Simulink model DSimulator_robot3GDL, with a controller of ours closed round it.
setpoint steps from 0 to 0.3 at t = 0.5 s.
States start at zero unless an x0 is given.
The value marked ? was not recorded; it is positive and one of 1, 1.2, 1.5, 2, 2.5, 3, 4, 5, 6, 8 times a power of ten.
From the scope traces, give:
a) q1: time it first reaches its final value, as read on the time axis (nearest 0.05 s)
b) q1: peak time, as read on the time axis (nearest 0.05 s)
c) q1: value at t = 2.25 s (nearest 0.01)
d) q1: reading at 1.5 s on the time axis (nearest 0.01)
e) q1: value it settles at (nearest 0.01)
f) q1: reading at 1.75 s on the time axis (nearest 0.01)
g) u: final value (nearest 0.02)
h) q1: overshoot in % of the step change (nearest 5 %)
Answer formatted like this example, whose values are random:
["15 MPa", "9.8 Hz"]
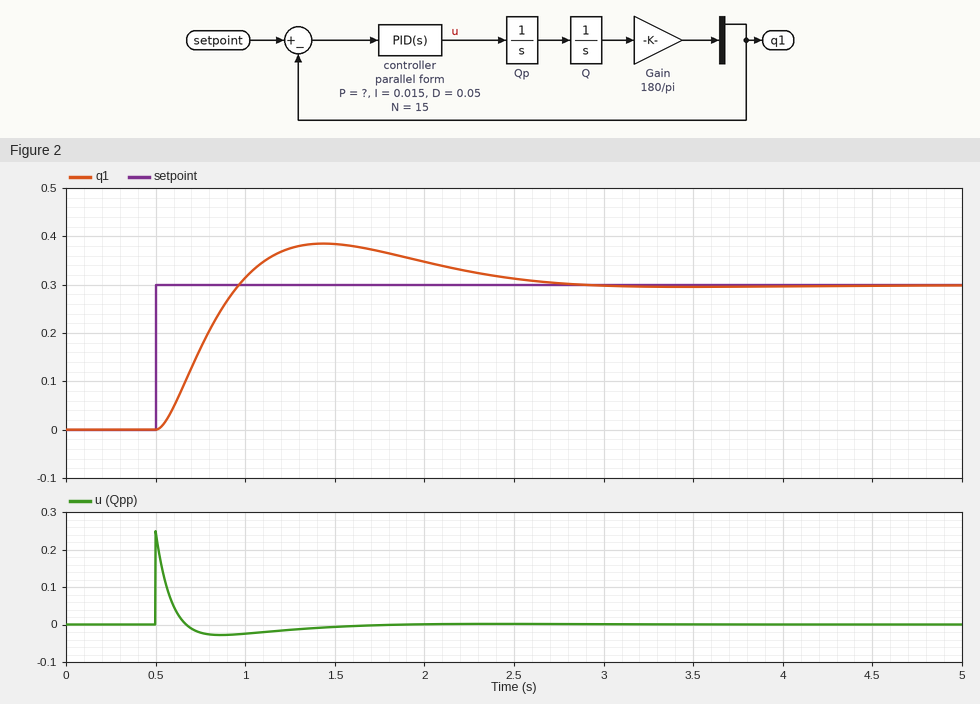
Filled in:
["0.95 s", "1.45 s", "0.33", "0.38", "0.30", "0.37", "0.00", "30 %"]
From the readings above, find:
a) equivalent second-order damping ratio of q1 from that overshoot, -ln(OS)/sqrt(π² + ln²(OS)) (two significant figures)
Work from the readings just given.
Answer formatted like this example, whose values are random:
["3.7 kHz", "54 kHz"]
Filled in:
["0.36"]
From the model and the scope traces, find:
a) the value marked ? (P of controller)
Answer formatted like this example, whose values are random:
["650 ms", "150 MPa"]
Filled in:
["0.08"]
